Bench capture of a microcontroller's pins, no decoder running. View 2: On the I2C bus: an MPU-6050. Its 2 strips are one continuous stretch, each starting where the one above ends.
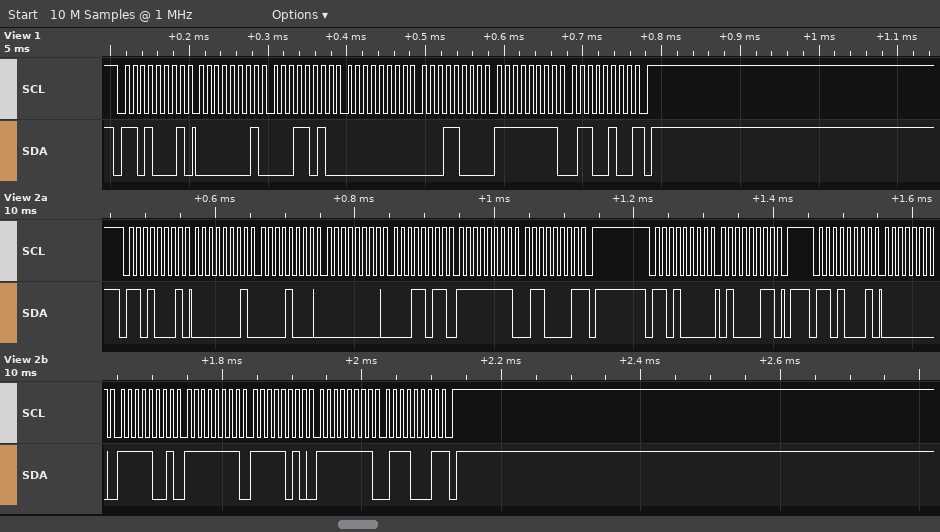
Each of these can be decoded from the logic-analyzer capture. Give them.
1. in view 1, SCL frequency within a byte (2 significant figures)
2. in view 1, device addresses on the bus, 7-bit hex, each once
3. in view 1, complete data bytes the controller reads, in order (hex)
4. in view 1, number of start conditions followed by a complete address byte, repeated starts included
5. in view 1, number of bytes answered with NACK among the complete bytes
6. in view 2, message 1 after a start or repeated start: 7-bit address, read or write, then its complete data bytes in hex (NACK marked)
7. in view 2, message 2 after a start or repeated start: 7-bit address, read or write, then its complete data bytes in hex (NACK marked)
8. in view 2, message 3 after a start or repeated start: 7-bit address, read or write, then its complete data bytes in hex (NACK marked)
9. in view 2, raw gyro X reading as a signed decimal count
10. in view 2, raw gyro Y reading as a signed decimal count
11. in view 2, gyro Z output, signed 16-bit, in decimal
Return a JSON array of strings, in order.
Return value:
["100 kHz", "0x68", "01 1A 00 18 FF 64", "1", "1", "0x68 read: 01 08 00 1B FF 61 NACK", "0x68 write: 43", "0x68 read: 00 F9 FF FA FF 71 NACK", "249", "-6", "-143"]
